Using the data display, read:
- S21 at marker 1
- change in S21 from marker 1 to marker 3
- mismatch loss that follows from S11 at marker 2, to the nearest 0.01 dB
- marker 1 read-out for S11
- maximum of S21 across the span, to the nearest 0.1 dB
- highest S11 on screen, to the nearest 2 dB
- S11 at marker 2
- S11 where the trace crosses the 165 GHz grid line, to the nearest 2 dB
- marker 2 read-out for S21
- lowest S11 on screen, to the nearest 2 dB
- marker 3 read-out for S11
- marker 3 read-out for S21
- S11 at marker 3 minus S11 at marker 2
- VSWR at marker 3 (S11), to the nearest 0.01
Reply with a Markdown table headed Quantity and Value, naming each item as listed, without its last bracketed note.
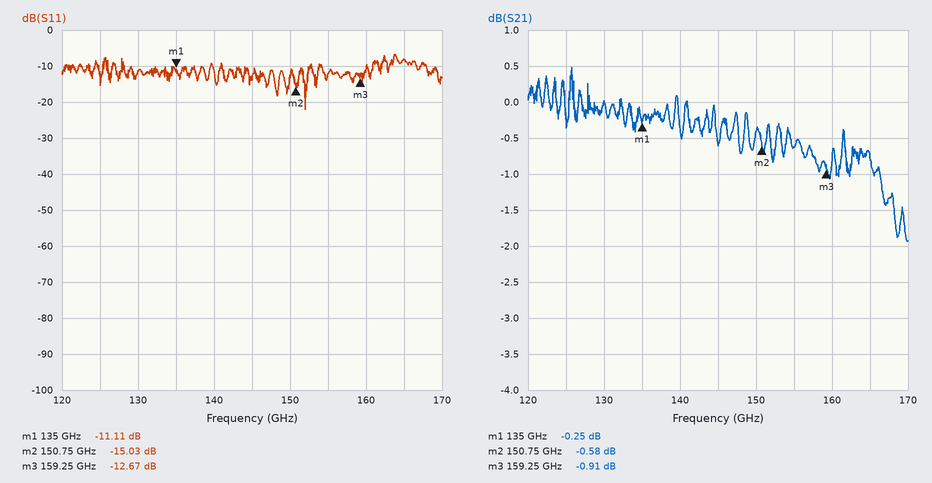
| Quantity | Value |
|---|---|
| S21 at marker 1 | -0.25 dB |
| change in S21 from marker 1 to marker 3 | -0.66 dB |
| mismatch loss that follows from S11 at marker 2, to the nearest 0.01 dB | 0.14 dB |
| marker 1 read-out for S11 | -11.11 dB |
| maximum of S21 across the span, to the nearest 0.1 dB | 0.5 dB |
| highest S11 on screen, to the nearest 2 dB | -6 dB |
| S11 at marker 2 | -15.03 dB |
| S11 where the trace crosses the 165 GHz grid line, to the nearest 2 dB | -8 dB |
| marker 2 read-out for S21 | -0.58 dB |
| lowest S11 on screen, to the nearest 2 dB | -22 dB |
| marker 3 read-out for S11 | -12.67 dB |
| marker 3 read-out for S21 | -0.91 dB |
| S11 at marker 3 minus S11 at marker 2 | 2.36 dB |
| VSWR at marker 3 (S11), to the nearest 0.01 | 1.61 |
